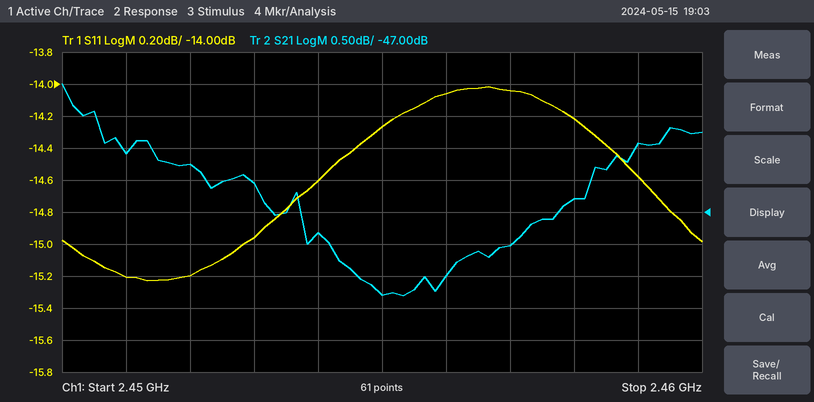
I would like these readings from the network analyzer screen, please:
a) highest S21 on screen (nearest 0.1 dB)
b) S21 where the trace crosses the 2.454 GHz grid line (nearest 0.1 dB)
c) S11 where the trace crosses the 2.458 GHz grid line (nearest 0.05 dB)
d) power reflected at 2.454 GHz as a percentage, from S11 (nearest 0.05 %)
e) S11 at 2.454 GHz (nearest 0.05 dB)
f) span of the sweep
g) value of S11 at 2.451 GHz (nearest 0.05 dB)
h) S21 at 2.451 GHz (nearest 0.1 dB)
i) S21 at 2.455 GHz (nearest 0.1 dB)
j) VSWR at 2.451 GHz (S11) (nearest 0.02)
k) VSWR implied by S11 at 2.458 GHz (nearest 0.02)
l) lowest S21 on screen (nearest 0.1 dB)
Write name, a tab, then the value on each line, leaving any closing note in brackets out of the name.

highest S21 on screen	-45.0 dB
S21 where the trace crosses the 2.454 GHz grid line	-47.3 dB
S11 where the trace crosses the 2.458 GHz grid line	-14.20 dB
power reflected at 2.454 GHz as a percentage, from S11	3.45 %
S11 at 2.454 GHz	-14.60 dB
span of the sweep	10 MHz
value of S11 at 2.451 GHz	-15.20 dB
S21 at 2.451 GHz	-46.1 dB
S21 at 2.455 GHz	-48.3 dB
VSWR at 2.451 GHz (S11)	1.42
VSWR implied by S11 at 2.458 GHz	1.48
lowest S21 on screen	-48.3 dB
